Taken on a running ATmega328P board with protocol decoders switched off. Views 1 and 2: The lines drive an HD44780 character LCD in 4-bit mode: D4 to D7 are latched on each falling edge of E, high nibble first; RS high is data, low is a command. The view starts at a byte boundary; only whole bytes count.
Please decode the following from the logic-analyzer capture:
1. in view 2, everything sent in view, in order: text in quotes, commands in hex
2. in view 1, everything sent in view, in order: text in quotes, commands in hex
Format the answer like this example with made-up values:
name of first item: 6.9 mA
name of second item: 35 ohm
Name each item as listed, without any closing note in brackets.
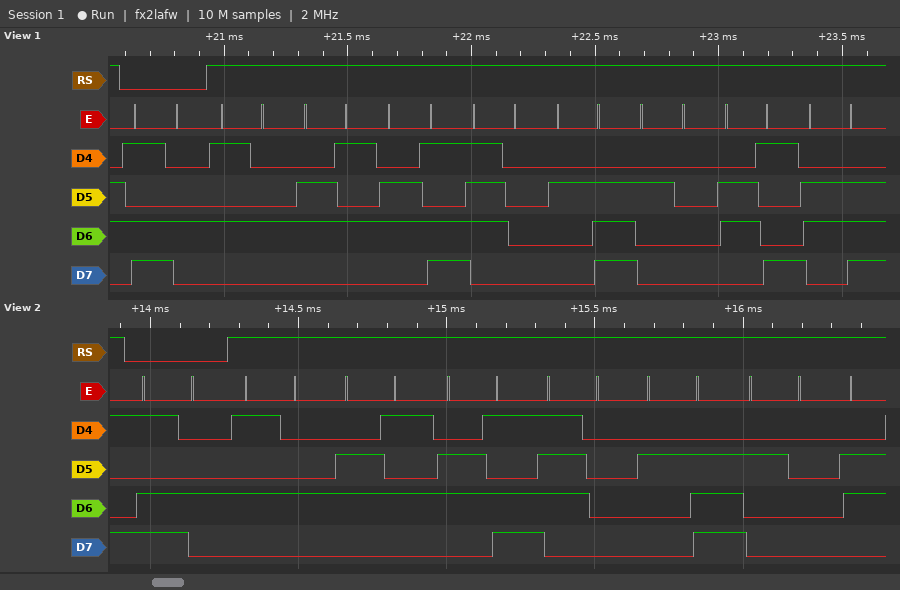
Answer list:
in view 2, everything sent in view, in order: text in quotes, commands in hex: 0xD4 "Temp. "
in view 1, everything sent in view, in order: text in quotes, commands in hex: 0xD4 "Temp. in"
